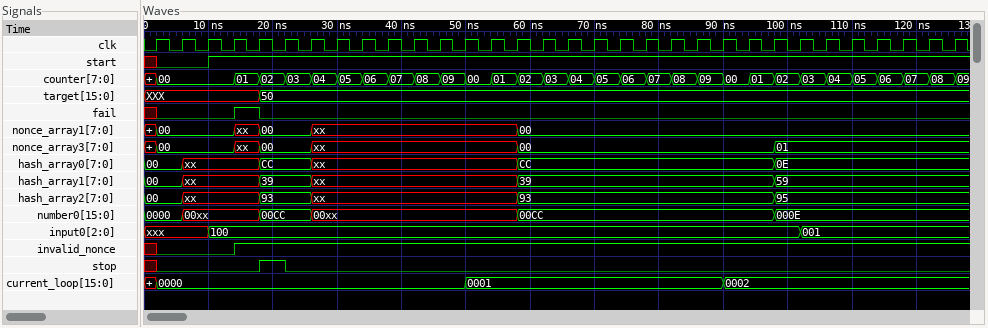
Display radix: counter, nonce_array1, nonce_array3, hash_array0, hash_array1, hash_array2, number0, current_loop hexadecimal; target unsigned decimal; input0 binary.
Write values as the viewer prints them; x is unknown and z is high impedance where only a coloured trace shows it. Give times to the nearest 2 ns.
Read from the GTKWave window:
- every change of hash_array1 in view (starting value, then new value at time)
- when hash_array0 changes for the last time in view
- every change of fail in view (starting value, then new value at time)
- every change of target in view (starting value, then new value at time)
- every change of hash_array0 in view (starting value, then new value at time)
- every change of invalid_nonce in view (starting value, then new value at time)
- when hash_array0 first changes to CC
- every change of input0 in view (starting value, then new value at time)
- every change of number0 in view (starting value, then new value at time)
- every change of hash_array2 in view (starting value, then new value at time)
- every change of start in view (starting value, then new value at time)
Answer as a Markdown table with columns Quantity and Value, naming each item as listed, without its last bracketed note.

| Quantity | Value |
|---|---|
| every change of hash_array1 in view | 00, xx at 6 ns, 39 at 18 ns, xx at 26 ns, 39 at 58 ns, 59 at 98 ns |
| when hash_array0 changes for the last time in view | 98 ns |
| every change of fail in view | x, 0 at 2 ns, 1 at 14 ns, 0 at 18 ns |
| every change of target in view | XXX, 50 at 18 ns |
| every change of hash_array0 in view | 00, xx at 6 ns, CC at 18 ns, xx at 26 ns, CC at 58 ns, 0E at 98 ns |
| every change of invalid_nonce in view | x, 0 at 2 ns, 1 at 14 ns |
| when hash_array0 first changes to CC | 18 ns |
| every change of input0 in view | xxx, 100 at 10 ns, 001 at 102 ns |
| every change of number0 in view | 0000, 00xx at 6 ns, 00CC at 18 ns, 00xx at 26 ns, 00CC at 58 ns, 000E at 98 ns |
| every change of hash_array2 in view | 00, xx at 6 ns, 93 at 18 ns, xx at 26 ns, 93 at 58 ns, 95 at 98 ns |
| every change of start in view | x, 0 at 2 ns, 1 at 10 ns |
